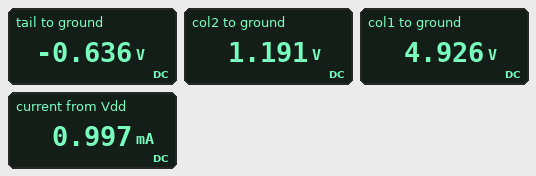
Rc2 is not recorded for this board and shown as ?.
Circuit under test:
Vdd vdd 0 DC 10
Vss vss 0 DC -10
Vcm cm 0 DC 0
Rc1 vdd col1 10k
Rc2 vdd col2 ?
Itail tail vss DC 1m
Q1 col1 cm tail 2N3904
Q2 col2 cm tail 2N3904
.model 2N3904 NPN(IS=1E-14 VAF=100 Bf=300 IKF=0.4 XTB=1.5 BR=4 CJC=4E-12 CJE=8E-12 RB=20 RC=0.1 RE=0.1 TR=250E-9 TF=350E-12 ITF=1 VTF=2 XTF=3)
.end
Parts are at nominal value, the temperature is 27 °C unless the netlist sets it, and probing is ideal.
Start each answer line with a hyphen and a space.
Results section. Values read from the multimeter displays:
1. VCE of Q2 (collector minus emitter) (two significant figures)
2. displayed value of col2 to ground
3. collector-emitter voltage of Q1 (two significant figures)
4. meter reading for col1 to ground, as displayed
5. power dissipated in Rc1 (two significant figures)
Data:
- 1.8 V
- 1.191 V
- 5.6 V
- 4.926 V
- 2.6 mW
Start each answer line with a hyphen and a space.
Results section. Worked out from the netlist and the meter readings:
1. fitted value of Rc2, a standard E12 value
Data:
- 18 kΩ
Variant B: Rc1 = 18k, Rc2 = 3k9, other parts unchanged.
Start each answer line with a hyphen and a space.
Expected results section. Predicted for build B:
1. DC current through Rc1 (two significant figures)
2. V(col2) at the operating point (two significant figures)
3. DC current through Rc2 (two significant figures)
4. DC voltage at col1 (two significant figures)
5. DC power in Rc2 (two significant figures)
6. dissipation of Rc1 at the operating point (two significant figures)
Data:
- 480 µA
- 8.0 V
- 510 µA
- 1.3 V
- 1.0 mW
- 4.2 mW
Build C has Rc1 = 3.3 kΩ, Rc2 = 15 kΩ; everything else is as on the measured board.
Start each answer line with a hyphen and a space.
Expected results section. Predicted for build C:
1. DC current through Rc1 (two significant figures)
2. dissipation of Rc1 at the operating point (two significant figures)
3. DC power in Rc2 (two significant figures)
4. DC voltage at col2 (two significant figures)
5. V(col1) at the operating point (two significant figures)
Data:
- 510 µA
- 860 µW
- 3.5 mW
- 2.7 V
- 8.3 V
